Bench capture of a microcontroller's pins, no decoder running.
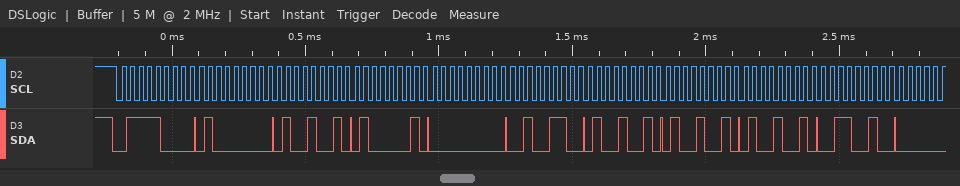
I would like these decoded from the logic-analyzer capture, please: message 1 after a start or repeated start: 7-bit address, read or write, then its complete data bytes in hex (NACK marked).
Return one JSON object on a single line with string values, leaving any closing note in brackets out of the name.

{"message 1 after a start or repeated start: 7-bit address, read or write, then its complete data bytes in hex": "0x3C write: 40 49 41 00 26 49 49 49 32"}
